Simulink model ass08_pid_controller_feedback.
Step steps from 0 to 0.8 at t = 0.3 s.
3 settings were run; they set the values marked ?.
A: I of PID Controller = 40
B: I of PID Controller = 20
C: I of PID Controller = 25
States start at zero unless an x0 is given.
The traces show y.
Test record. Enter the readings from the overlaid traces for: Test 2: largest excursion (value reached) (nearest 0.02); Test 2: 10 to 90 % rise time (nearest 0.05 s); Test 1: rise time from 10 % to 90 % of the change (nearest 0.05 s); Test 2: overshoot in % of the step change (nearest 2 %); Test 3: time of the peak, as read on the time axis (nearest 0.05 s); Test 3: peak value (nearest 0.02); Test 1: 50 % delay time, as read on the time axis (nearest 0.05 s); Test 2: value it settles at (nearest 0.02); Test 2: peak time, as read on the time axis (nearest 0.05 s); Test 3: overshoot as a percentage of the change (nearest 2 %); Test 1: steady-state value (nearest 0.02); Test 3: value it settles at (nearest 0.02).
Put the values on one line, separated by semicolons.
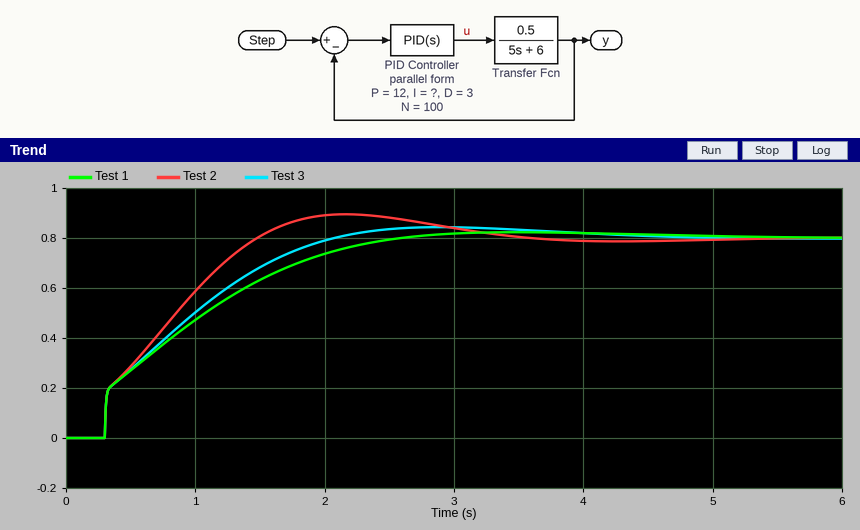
0.90; 0.95 s; 1.60 s; 12 %; 2.90 s; 0.84; 0.80 s; 0.80; 2.15 s; 6 %; 0.80; 0.80
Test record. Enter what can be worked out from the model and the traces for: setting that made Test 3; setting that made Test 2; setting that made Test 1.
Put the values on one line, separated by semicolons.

C; A; B
